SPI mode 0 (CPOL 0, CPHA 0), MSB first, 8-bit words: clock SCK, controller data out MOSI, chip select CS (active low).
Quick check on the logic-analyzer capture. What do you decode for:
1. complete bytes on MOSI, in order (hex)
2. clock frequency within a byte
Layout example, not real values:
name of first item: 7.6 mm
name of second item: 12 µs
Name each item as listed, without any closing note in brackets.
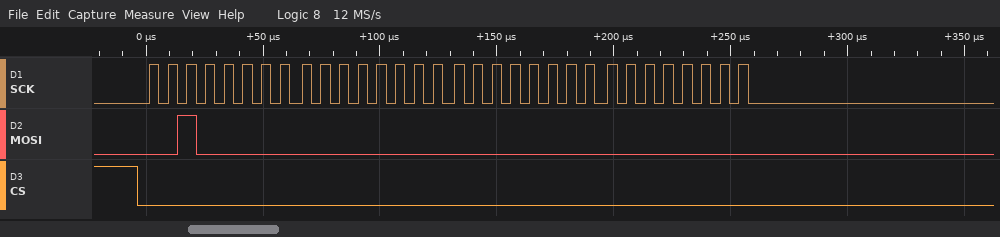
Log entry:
complete bytes on MOSI, in order: 20 00 00 00
clock frequency within a byte: 125 kHz
